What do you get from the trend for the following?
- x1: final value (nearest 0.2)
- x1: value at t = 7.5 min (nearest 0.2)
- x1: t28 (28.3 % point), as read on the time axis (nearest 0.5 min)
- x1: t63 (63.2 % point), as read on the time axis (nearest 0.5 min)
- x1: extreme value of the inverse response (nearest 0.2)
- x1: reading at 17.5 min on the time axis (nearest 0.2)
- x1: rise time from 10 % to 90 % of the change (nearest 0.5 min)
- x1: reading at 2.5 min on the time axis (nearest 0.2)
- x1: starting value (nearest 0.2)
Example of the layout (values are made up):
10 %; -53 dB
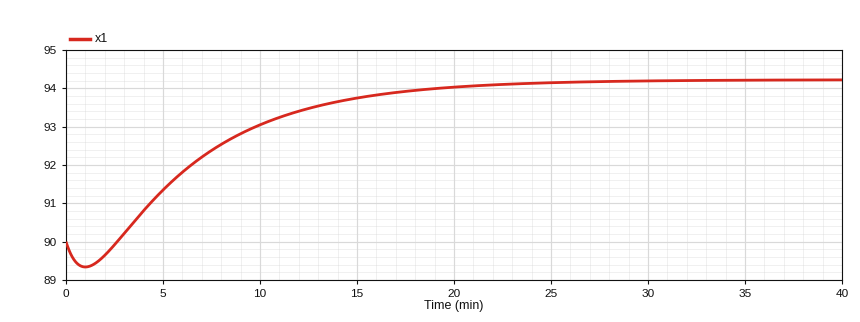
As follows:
94.2; 92.4; 4.5 min; 8.5 min; 89.4; 94.0; 12.5 min; 90.0; 90.0
